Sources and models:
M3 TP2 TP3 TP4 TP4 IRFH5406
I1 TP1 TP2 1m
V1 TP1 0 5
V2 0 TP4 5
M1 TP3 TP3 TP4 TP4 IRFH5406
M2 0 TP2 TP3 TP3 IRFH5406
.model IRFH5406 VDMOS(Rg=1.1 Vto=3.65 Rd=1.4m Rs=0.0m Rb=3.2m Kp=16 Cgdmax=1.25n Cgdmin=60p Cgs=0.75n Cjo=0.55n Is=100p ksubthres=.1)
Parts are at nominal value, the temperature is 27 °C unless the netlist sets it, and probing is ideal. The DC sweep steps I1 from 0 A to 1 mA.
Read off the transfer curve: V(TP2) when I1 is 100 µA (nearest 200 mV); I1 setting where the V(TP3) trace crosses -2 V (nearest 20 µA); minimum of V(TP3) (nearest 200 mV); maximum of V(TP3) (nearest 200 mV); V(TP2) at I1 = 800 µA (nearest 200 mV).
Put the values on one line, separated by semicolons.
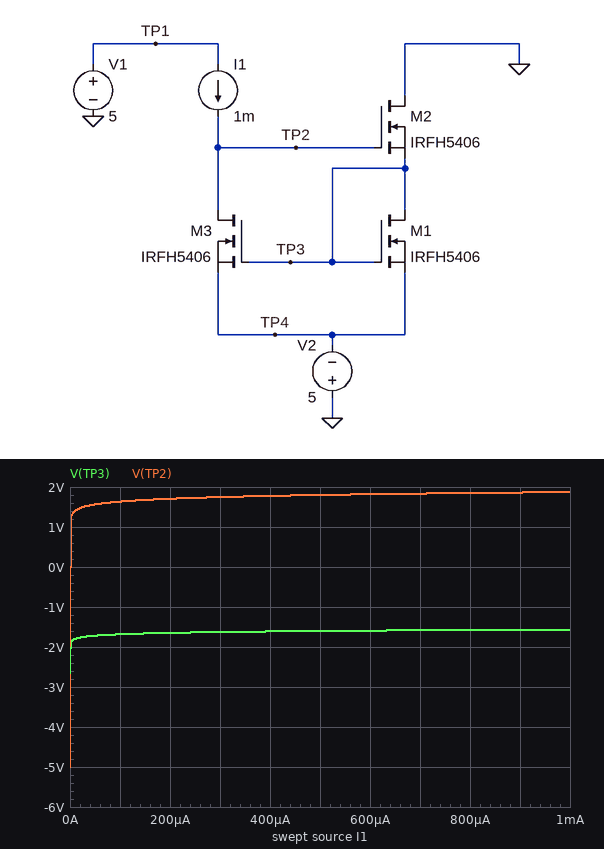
1.6 V; 0 A; -2.6 V; -1.6 V; 1.8 V
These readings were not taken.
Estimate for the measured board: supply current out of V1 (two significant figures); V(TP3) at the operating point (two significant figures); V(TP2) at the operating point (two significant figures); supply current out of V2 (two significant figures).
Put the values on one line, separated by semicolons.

1.0 mA; -1.6 V; 1.9 V; 2.0 mA
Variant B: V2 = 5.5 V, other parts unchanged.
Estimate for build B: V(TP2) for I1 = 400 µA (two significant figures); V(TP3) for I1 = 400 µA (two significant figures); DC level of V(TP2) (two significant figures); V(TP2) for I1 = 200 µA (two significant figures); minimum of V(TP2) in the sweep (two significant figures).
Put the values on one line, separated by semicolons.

1.3 V; -2.1 V; 1.4 V; 1.2 V; -5.5 V
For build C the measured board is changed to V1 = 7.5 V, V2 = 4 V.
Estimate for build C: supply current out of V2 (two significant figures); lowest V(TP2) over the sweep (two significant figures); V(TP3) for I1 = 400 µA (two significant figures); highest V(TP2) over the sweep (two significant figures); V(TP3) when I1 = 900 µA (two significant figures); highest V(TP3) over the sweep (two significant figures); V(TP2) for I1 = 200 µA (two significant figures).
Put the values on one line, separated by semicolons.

2.0 mA; -4.0 V; -610 mV; 2.9 V; -570 mV; -560 mV; 2.7 V
